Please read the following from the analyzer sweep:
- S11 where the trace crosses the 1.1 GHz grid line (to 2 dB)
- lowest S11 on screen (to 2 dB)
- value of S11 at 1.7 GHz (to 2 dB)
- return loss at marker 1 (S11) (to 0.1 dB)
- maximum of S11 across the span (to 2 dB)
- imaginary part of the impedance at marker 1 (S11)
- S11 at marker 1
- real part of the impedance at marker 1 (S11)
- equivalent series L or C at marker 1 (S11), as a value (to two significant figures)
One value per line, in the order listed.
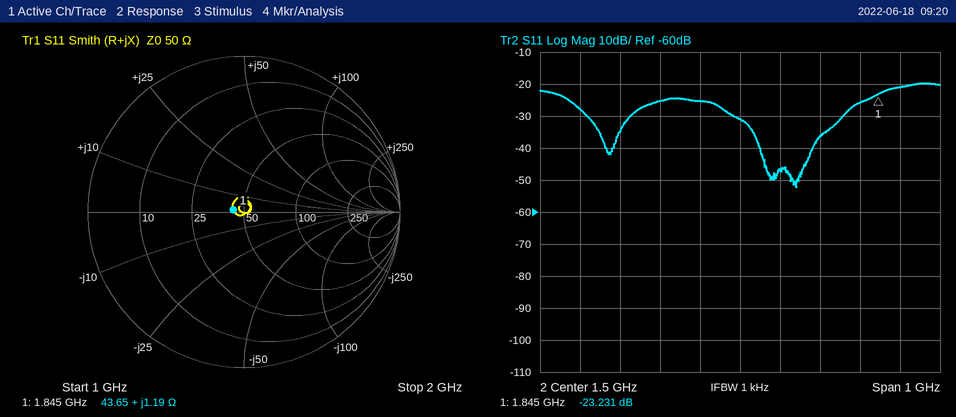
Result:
-28 dB
-52 dB
-36 dB
23.2 dB
-20 dB
+1.19 Ω
-23.231 dB
43.65 Ω
100 pH
